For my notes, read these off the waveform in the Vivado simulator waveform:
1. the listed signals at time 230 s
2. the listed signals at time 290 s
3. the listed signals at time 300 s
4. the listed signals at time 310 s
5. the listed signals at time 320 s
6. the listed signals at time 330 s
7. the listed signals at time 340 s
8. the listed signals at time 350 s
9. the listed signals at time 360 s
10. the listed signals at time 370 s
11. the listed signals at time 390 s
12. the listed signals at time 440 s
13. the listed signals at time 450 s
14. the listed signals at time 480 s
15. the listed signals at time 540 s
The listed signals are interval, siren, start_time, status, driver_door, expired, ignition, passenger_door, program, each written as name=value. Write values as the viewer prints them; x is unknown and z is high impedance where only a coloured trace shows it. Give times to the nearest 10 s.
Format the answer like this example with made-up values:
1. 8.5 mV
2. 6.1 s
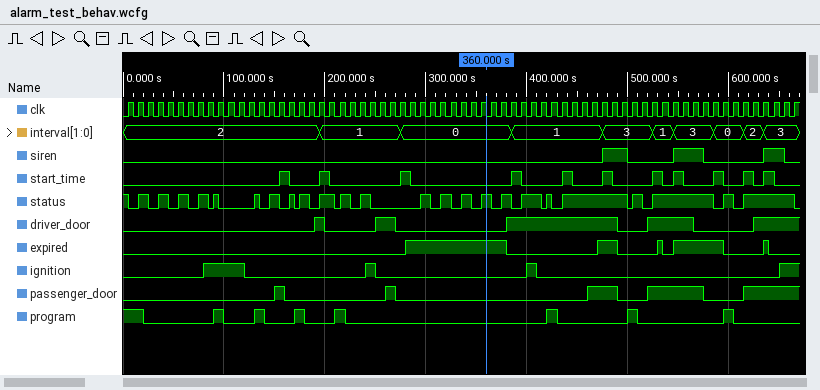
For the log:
1. interval=1, siren=0, start_time=0, status=0, driver_door=0, expired=0, ignition=0, passenger_door=0, program=0
2. interval=0, siren=0, start_time=0, status=0, driver_door=0, expired=1, ignition=0, passenger_door=0, program=0
3. interval=0, siren=0, start_time=0, status=1, driver_door=0, expired=1, ignition=0, passenger_door=0, program=0
4. interval=0, siren=0, start_time=0, status=0, driver_door=0, expired=1, ignition=0, passenger_door=0, program=0
5. interval=0, siren=0, start_time=0, status=1, driver_door=0, expired=1, ignition=0, passenger_door=0, program=0
6. interval=0, siren=0, start_time=0, status=0, driver_door=0, expired=1, ignition=0, passenger_door=0, program=0
7. interval=0, siren=0, start_time=0, status=1, driver_door=0, expired=1, ignition=0, passenger_door=0, program=0
8. interval=0, siren=0, start_time=0, status=0, driver_door=0, expired=1, ignition=0, passenger_door=0, program=0
9. interval=0, siren=0, start_time=0, status=1, driver_door=0, expired=1, ignition=0, passenger_door=0, program=0
10. interval=0, siren=0, start_time=0, status=0, driver_door=0, expired=1, ignition=0, passenger_door=0, program=0
11. interval=1, siren=0, start_time=1, status=0, driver_door=1, expired=0, ignition=0, passenger_door=0, program=0
12. interval=1, siren=0, start_time=1, status=1, driver_door=1, expired=0, ignition=0, passenger_door=0, program=0
13. interval=1, siren=0, start_time=0, status=1, driver_door=1, expired=0, ignition=0, passenger_door=0, program=0
14. interval=3, siren=1, start_time=1, status=1, driver_door=1, expired=1, ignition=0, passenger_door=1, program=0
15. interval=1, siren=0, start_time=0, status=1, driver_door=1, expired=0, ignition=0, passenger_door=1, program=0
